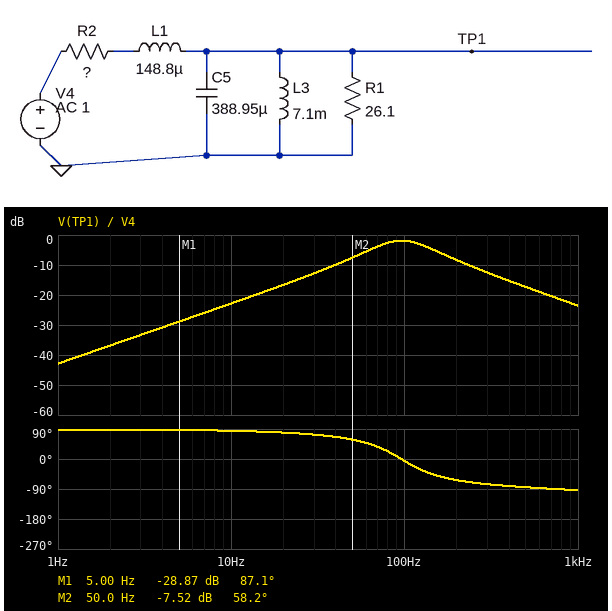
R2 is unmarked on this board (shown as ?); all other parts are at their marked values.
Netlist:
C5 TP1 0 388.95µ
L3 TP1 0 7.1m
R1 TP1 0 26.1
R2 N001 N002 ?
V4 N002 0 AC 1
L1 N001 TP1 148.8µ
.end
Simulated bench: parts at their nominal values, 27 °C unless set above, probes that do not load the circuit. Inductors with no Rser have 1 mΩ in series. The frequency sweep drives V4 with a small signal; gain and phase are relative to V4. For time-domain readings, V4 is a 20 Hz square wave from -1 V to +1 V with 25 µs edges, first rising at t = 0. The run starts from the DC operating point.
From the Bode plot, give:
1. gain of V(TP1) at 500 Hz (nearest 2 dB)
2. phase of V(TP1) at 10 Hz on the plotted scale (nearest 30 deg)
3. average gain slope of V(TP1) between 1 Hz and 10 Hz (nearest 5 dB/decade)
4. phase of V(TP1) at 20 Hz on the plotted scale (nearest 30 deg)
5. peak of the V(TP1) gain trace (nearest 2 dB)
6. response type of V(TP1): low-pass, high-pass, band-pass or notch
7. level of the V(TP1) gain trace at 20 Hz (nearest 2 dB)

-18 dB
90 deg
20 dB/decade
90 deg
-2 dB
band-pass
-16 dB
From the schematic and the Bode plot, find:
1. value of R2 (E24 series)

6.2 Ω
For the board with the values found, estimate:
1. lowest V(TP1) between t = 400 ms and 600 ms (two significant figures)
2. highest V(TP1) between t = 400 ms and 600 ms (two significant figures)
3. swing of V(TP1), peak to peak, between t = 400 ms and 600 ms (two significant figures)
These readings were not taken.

-810 mV
810 mV
1.6 V
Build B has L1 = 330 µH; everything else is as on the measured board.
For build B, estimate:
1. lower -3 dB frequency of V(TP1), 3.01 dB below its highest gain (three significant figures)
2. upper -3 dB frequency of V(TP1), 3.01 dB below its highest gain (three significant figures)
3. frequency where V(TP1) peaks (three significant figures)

63.7 Hz
147 Hz
96.9 Hz
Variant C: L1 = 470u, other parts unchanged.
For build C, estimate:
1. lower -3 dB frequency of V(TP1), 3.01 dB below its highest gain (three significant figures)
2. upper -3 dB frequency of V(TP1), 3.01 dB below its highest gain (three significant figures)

63.9 Hz
148 Hz
